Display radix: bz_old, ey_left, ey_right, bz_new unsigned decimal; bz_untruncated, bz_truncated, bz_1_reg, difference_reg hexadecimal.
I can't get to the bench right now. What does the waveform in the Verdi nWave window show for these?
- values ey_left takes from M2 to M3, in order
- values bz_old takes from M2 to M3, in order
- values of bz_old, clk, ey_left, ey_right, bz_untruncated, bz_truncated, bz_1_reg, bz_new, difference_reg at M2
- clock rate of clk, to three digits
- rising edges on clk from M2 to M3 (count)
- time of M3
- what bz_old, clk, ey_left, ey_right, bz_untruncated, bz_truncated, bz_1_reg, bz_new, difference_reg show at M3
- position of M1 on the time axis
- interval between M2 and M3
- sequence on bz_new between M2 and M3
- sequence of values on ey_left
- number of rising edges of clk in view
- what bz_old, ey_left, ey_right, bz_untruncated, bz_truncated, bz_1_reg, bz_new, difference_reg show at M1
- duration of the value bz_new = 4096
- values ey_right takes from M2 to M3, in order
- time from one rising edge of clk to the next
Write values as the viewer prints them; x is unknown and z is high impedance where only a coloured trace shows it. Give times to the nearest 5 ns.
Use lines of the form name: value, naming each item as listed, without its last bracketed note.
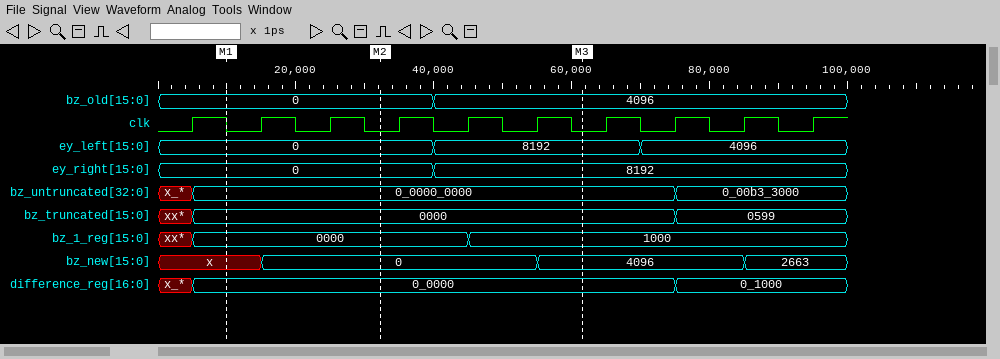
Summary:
values ey_left takes from M2 to M3, in order: 0, 8192
values bz_old takes from M2 to M3, in order: 0, 4096
values of bz_old, clk, ey_left, ey_right, bz_untruncated, bz_truncated, bz_1_reg, bz_new, difference_reg at M2: bz_old=0, clk=0, ey_left=0, ey_right=0, bz_untruncated=0_0000_0000, bz_truncated=0000, bz_1_reg=0000, bz_new=0, difference_reg=0_0000
clock rate of clk, to three digits: 100 MHz
rising edges on clk from M2 to M3: 3
time of M3: 60 ns
what bz_old, clk, ey_left, ey_right, bz_untruncated, bz_truncated, bz_1_reg, bz_new, difference_reg show at M3: bz_old=4096, clk=0, ey_left=8192, ey_right=8192, bz_untruncated=0_0000_0000, bz_truncated=0000, bz_1_reg=1000, bz_new=4096, difference_reg=0_0000
position of M1 on the time axis: 10 ns
interval between M2 and M3: 30 ns
sequence on bz_new between M2 and M3: 0, 4096
sequence of values on ey_left: 0, 8192, 4096
number of rising edges of clk in view: 10
what bz_old, ey_left, ey_right, bz_untruncated, bz_truncated, bz_1_reg, bz_new, difference_reg show at M1: bz_old=0, ey_left=0, ey_right=0, bz_untruncated=0_0000_0000, bz_truncated=0000, bz_1_reg=0000, bz_new=x, difference_reg=0_0000
duration of the value bz_new = 4096: 30 ns
values ey_right takes from M2 to M3, in order: 0, 8192
time from one rising edge of clk to the next: 10 ns
